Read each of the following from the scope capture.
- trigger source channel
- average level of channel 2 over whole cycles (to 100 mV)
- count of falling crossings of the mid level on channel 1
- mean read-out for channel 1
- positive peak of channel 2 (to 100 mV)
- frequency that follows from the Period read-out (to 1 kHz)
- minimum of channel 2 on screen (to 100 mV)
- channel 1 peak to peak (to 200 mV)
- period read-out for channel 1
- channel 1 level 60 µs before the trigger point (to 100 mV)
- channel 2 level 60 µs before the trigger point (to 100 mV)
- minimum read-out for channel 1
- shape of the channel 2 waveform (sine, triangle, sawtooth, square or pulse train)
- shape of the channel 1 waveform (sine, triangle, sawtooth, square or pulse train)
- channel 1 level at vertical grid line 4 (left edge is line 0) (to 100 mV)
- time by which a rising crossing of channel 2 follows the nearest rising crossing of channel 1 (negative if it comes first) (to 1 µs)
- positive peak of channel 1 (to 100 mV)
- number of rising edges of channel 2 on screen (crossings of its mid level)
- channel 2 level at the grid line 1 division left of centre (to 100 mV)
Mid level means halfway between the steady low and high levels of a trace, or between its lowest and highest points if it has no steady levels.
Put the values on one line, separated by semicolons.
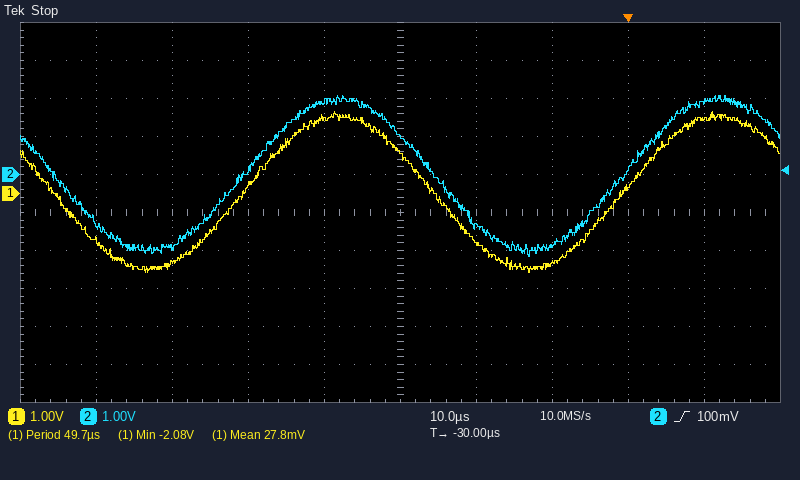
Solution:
channel 2; 0.0 V; 2; 27.8 mV; 2.1 V; 20 kHz; -2.2 V; 4.2 V; 49.7 µs; -1.8 V; -1.9 V; -2.08 V; sine; sine; 2.0 V; 0 µs; 2.2 V; 2; 1.9 V
